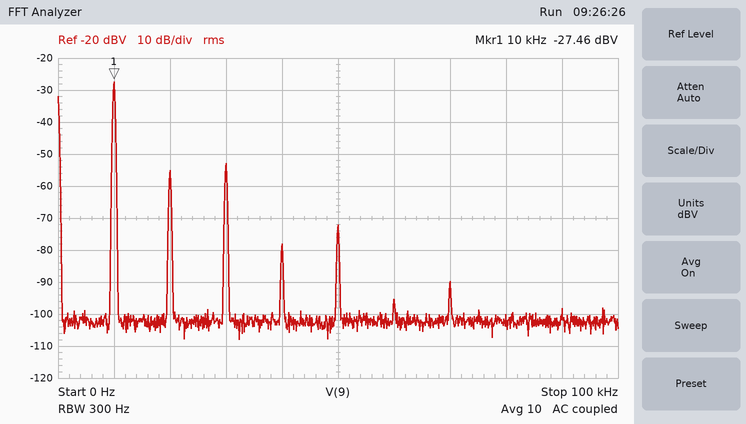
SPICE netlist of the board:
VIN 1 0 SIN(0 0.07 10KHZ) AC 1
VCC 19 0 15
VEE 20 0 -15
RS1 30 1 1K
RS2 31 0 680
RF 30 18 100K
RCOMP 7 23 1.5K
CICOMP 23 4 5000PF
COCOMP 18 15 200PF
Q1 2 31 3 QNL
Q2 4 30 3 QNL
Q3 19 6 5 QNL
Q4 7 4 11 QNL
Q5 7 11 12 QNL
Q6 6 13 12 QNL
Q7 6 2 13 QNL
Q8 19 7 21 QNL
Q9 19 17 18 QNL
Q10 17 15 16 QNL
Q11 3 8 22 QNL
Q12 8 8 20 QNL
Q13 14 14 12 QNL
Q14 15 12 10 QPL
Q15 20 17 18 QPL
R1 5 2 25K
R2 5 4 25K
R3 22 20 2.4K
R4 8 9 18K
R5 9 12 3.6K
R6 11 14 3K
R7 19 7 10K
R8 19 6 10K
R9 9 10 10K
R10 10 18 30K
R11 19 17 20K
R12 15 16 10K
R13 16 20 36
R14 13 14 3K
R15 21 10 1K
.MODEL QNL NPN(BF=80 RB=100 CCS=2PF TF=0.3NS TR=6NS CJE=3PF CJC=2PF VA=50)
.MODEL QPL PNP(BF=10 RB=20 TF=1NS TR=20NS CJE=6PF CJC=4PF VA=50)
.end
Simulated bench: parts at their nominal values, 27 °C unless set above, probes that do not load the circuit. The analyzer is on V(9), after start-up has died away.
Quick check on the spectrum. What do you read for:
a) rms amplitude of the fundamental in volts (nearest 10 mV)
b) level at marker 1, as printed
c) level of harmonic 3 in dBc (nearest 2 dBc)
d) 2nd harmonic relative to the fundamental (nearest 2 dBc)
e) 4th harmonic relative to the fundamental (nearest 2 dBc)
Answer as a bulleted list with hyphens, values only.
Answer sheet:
- 40 mV
- -27.46 dBV
- -26 dBc
- -28 dBc
- -50 dBc
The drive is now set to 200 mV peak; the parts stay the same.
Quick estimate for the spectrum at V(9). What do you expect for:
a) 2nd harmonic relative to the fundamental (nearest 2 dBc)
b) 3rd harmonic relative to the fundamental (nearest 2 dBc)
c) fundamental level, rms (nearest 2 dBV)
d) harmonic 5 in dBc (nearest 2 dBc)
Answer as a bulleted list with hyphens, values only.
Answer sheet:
- -22 dBc
- -16 dBc
- -24 dBV
- -26 dBc
